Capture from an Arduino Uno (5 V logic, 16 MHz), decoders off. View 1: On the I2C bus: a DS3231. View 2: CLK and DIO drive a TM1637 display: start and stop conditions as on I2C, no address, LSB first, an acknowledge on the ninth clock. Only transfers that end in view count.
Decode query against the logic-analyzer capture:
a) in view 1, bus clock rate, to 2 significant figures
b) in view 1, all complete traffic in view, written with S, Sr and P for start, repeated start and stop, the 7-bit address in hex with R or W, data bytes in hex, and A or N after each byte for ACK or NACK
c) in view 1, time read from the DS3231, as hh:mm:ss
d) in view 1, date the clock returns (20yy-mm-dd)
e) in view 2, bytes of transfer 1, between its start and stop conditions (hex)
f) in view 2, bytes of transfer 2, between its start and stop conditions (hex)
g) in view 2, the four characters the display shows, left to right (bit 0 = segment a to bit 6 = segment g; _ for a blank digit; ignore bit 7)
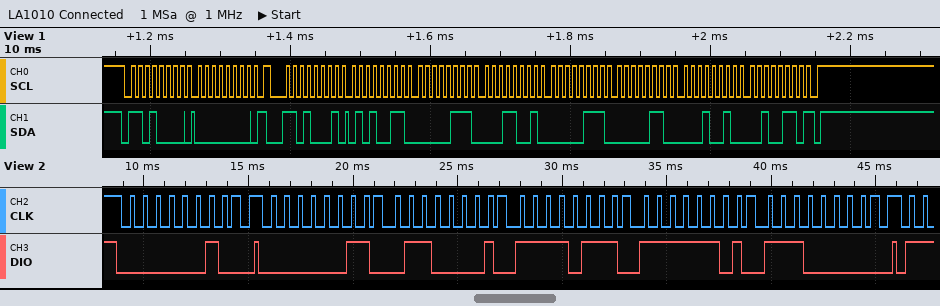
100 kHz
S 68W A 00 A Sr 68R A 53 A 07 A 19 A 07 A 06 A 12 A 26 N P
19:07:53
2026-12-06
40
C0 86 EF BF 07
1907
